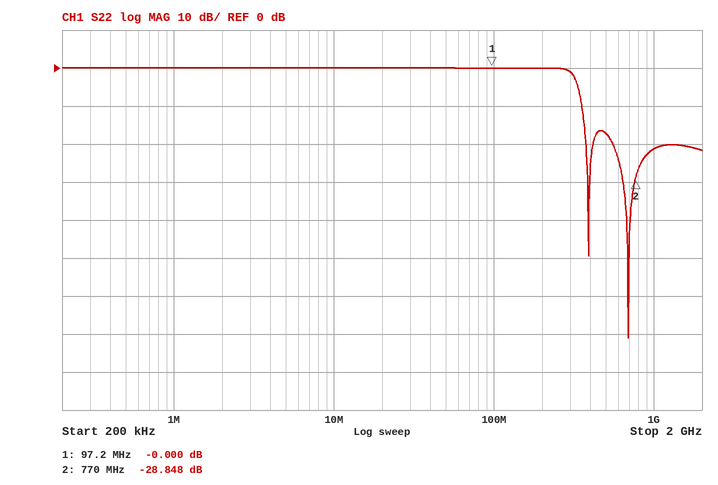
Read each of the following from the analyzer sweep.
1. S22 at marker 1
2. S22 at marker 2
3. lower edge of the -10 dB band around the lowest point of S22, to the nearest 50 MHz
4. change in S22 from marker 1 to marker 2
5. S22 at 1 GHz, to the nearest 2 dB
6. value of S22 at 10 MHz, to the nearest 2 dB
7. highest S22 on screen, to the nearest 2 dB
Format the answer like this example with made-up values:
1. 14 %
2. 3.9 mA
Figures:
1. -0.000 dB
2. -28.848 dB
3. 350 MHz
4. -28.848 dB
5. -22 dB
6. 0 dB
7. 0 dB
